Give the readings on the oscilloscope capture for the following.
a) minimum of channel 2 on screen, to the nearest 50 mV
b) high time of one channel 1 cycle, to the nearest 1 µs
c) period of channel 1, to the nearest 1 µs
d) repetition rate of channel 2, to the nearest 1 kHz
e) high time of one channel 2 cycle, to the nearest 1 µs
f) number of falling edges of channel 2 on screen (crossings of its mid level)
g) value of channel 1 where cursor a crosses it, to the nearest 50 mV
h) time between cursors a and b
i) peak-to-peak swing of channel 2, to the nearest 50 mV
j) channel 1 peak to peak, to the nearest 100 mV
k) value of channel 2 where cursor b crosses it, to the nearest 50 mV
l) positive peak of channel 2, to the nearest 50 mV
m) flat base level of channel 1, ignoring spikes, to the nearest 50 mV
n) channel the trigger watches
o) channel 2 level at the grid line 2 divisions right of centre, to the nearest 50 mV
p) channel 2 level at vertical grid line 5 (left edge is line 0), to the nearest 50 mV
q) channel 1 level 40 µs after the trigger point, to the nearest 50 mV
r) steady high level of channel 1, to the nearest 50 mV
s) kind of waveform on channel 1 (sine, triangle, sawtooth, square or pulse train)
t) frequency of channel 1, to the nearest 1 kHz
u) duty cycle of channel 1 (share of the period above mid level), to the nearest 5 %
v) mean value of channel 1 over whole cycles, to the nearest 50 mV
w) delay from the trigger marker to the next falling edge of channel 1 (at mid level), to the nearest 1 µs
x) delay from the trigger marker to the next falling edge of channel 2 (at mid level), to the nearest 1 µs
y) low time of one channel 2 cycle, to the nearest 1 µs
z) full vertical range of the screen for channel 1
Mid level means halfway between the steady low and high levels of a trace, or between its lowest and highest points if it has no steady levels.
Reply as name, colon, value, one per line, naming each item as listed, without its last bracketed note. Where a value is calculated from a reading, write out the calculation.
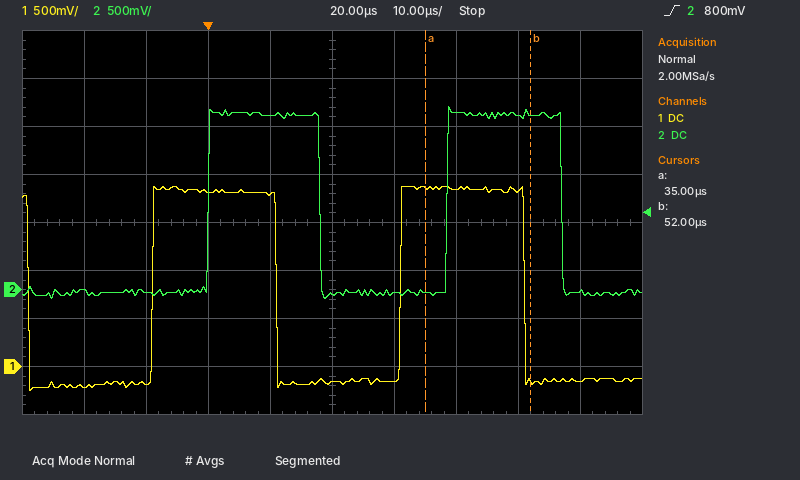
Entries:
minimum of channel 2 on screen, to the nearest 50 mV: -100 mV
high time of one channel 1 cycle, to the nearest 1 µs: 20 µs
period of channel 1, to the nearest 1 µs: 40 µs
repetition rate of channel 2, to the nearest 1 kHz: 26 kHz
high time of one channel 2 cycle, to the nearest 1 µs: 18 µs
number of falling edges of channel 2 on screen: 2
value of channel 1 where cursor a crosses it, to the nearest 50 mV: 1.85 V
time between cursors a and b: 52 µs − (35 µs) = 17 µs
peak-to-peak swing of channel 2, to the nearest 50 mV: 1.90 V − (-100 mV) = 2.00 V
channel 1 peak to peak, to the nearest 100 mV: 2.10 V
value of channel 2 where cursor b crosses it, to the nearest 50 mV: 1.85 V
positive peak of channel 2, to the nearest 50 mV: 1.90 V
flat base level of channel 1, ignoring spikes, to the nearest 50 mV: -150 mV
channel the trigger watches: channel 2
channel 2 level at the grid line 2 divisions right of centre, to the nearest 50 mV: 1.85 V
channel 2 level at vertical grid line 5 (left edge is line 0), to the nearest 50 mV: -50 mV
channel 1 level 40 µs after the trigger point, to the nearest 50 mV: 1.85 V
steady high level of channel 1, to the nearest 50 mV: 1.85 V
kind of waveform on channel 1: square
frequency of channel 1, to the nearest 1 kHz: 1 / 40 µs ≈ 25 kHz
duty cycle of channel 1 (share of the period above mid level), to the nearest 5 %: 20 µs / 40 µs ≈ 50 %
mean value of channel 1 over whole cycles, to the nearest 50 mV: -150 mV + 0.5 × (1.85 V − (-150 mV)) ≈ 850 mV
delay from the trigger marker to the next falling edge of channel 1 (at mid level), to the nearest 1 µs: 11 µs
delay from the trigger marker to the next falling edge of channel 2 (at mid level), to the nearest 1 µs: 18 µs
low time of one channel 2 cycle, to the nearest 1 µs: 20 µs
full vertical range of the screen for channel 1: 4 V
